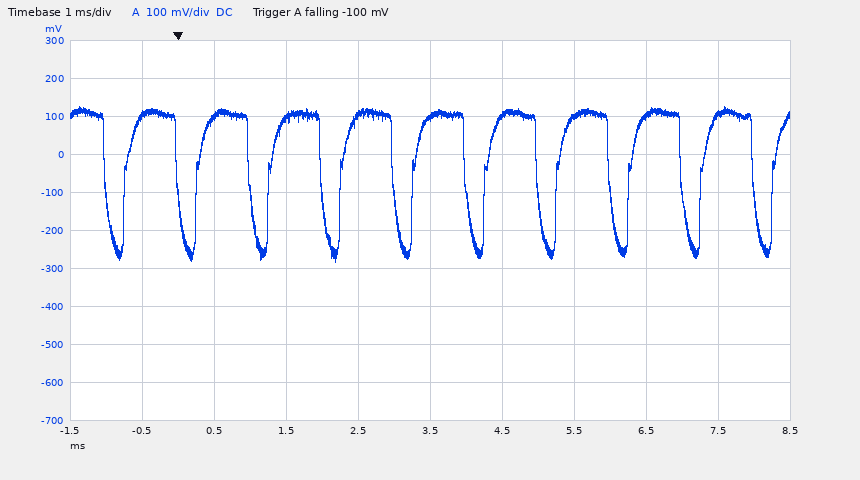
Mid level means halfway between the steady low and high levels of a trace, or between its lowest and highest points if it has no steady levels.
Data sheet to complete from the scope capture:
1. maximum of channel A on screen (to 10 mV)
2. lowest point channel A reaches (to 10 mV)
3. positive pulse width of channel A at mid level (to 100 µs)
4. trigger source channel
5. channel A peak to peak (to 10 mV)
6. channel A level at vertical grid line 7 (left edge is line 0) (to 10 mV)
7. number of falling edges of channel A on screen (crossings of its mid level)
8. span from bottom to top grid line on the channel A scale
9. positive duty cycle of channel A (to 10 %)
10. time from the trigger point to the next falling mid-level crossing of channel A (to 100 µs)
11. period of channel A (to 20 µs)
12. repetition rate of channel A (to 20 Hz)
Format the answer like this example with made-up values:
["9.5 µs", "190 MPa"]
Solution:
["130 mV", "-280 mV", "700 µs", "channel A", "410 mV", "100 mV", "10", "1 V", "70 %", "1.0 ms", "1.00 ms", "1.00 kHz"]
